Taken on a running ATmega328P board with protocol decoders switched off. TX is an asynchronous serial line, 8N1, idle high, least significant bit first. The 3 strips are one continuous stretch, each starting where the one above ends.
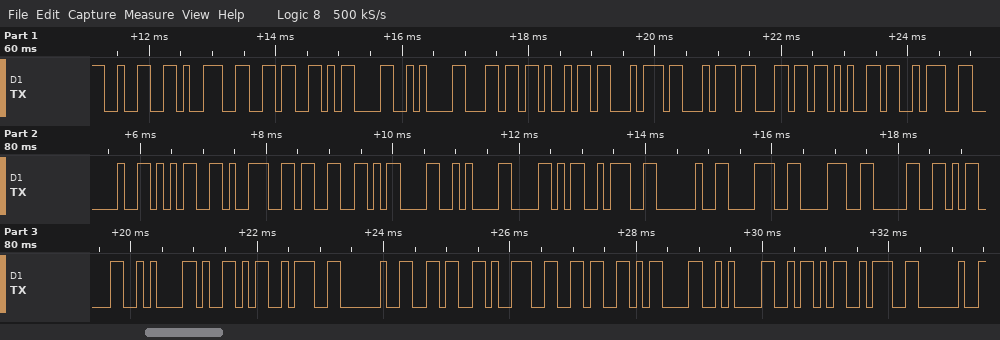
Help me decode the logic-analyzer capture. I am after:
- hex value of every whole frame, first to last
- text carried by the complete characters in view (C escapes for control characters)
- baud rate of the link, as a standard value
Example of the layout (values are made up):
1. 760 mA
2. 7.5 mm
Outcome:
1. 32 39 36 0D 0A 6C 69 74 74 6C 65 3A 20 35 39 33 0D 0A 58 3A 20 38 38 30 0D 0A 59 3A 20 36 39 36 0D 0A 5A 3A 20
2. "296\r\nlittle: 593\r\nX: 880\r\nY: 696\r\nZ: "
3. 9600 baud
